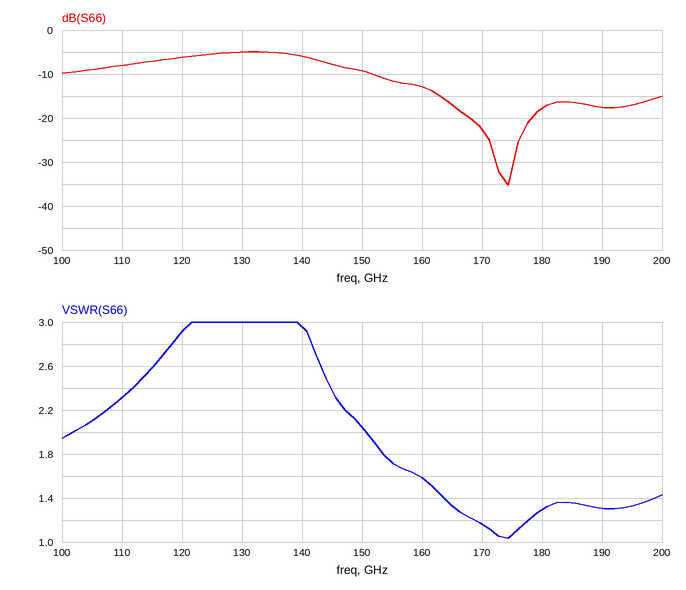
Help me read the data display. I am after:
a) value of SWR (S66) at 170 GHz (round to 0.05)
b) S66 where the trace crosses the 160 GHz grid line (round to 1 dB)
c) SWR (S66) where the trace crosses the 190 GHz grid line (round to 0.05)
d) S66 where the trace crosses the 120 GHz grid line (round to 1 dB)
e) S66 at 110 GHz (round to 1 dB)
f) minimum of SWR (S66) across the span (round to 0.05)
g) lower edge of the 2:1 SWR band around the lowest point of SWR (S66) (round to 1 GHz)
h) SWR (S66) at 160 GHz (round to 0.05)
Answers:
1.15
-13 dB
1.30
-6 dB
-8 dB
1.05
151 GHz
1.60
